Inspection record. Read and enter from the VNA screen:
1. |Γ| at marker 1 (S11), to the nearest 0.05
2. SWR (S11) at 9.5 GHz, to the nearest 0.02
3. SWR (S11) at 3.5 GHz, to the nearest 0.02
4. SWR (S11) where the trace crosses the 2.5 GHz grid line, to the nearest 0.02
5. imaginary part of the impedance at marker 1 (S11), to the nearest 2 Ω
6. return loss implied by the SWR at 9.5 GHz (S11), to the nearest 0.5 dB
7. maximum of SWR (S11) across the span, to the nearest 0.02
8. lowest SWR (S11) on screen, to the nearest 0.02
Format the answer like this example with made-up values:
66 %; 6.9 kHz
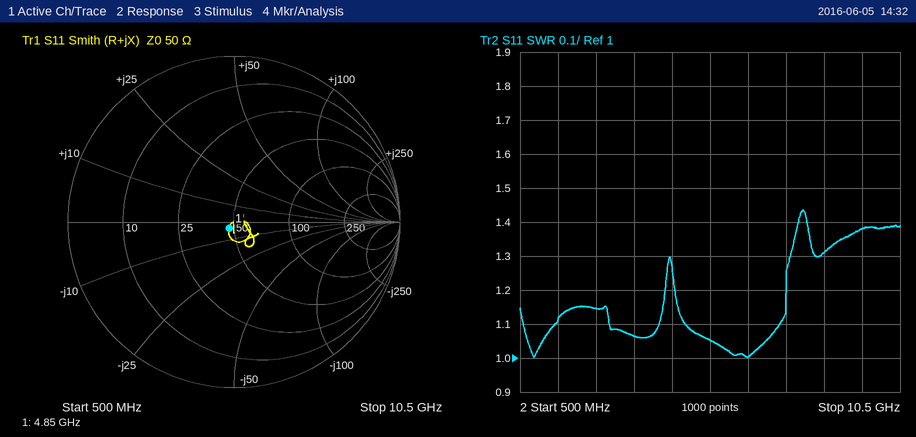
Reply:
0.05; 1.38; 1.06; 1.14; -4 Ω; 16.0 dB; 1.44; 1.00
